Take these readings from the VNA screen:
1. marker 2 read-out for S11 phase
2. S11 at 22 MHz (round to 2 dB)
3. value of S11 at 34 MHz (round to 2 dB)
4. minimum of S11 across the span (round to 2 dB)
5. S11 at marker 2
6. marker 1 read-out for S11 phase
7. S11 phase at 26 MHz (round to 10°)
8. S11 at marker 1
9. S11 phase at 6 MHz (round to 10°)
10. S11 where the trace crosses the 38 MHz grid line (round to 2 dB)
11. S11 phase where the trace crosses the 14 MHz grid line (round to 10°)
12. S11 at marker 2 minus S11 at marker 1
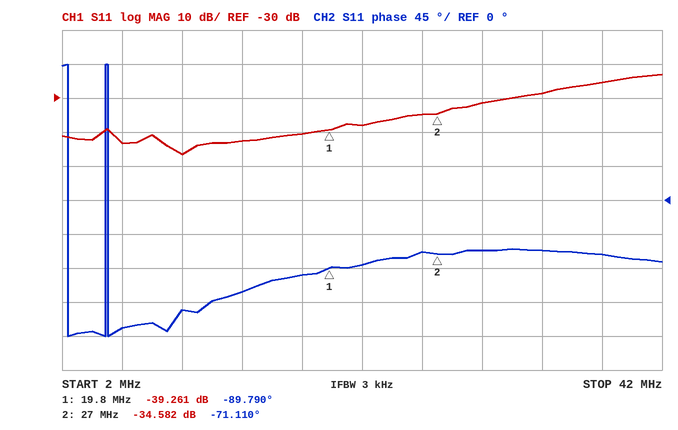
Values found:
-71.110°
-38 dB
-28 dB
-46 dB
-34.582 dB
-89.790°
-70°
-39.261 dB
-170°
-26 dB
-120°
4.679 dB
